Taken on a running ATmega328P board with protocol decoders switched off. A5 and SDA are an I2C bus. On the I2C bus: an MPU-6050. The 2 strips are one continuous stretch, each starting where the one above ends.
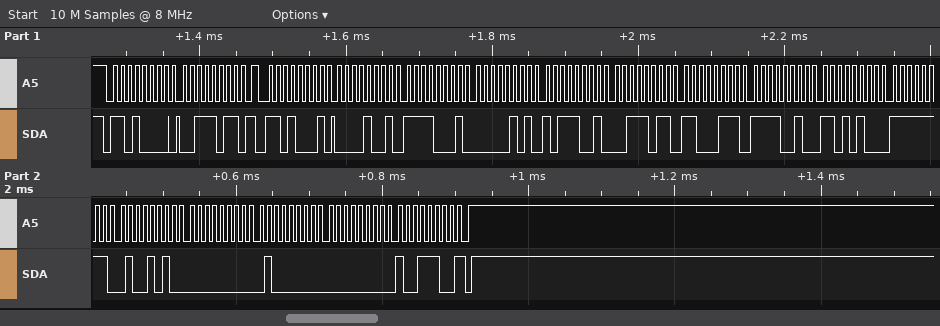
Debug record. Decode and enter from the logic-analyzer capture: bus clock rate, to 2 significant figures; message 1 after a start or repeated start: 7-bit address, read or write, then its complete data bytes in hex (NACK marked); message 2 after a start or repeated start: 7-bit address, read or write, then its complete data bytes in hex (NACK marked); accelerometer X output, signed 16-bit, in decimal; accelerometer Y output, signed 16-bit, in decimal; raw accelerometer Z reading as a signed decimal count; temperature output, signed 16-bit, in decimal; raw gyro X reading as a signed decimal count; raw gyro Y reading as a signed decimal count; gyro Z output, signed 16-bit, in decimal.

100 kHz
0x68 write: 3B
0x68 read: 09 F1 05 B9 3B C7 F2 D4 FF 4A 00 40 00 9C NACK
2545
1465
15303
-3372
-182
64
156
